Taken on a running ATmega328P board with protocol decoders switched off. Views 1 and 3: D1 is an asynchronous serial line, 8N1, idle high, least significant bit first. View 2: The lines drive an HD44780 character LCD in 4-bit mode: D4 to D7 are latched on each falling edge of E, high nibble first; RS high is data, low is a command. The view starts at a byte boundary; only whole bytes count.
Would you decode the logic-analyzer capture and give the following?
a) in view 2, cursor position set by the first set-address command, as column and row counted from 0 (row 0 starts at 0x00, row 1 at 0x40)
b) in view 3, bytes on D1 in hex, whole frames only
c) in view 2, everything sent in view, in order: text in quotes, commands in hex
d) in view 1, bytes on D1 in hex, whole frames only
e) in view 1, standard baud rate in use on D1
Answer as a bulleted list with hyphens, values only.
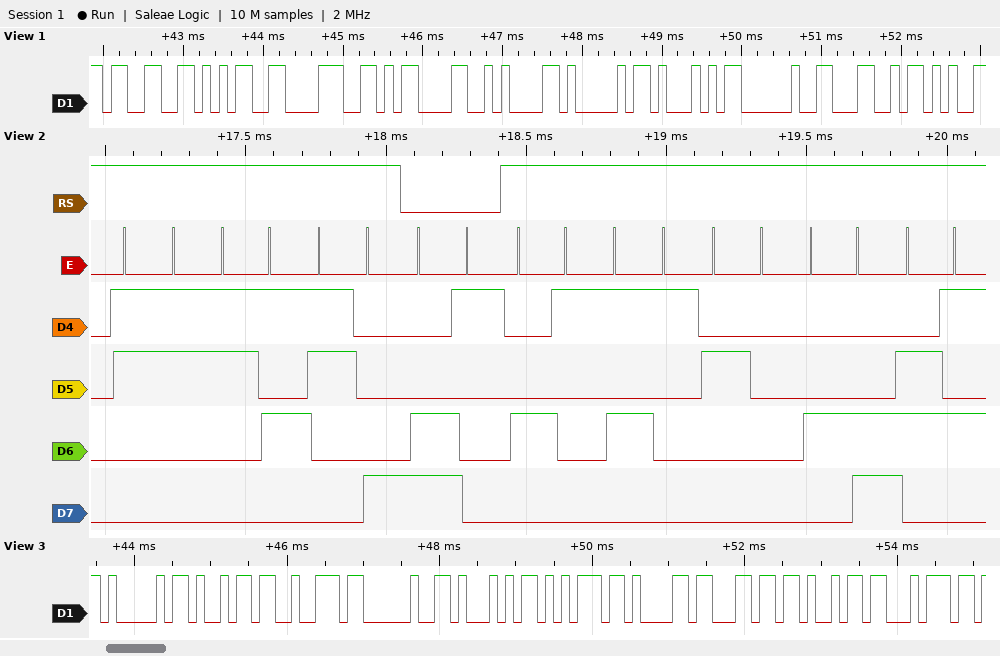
- column 1, row 1
- 41 69 72 20 51 75 61 6C 69 74
- "358" 0xC1 "AQ Le"
- 33 35 38 0D 0A 41 51 20 4C
- 9600 baud
